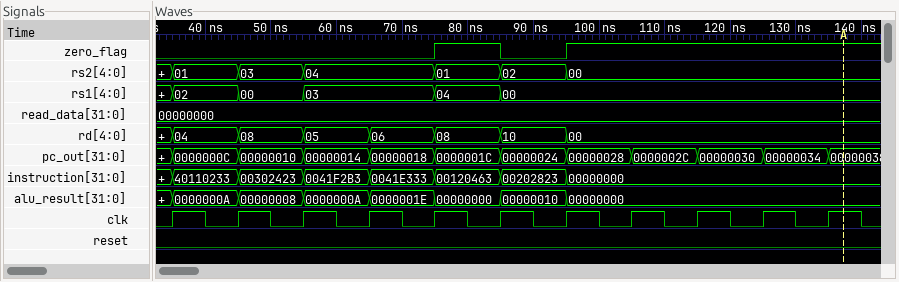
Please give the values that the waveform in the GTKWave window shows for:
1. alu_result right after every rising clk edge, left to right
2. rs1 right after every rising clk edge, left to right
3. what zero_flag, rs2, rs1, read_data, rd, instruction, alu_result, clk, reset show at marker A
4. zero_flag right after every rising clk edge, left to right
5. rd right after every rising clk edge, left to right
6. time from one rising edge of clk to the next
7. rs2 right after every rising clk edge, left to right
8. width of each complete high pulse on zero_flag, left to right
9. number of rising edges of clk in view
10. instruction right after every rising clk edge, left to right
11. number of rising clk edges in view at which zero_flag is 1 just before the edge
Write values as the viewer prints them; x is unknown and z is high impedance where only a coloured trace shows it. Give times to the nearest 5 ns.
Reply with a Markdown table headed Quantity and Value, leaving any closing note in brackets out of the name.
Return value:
| Quantity | Value |
|---|---|
| alu_result right after every rising clk edge, left to right | 0000000A, 00000008, 0000000A, 0000001E, 00000000, 00000010, 00000000, 00000000, 00000000, 00000000, 00000000 |
| rs1 right after every rising clk edge, left to right | 02, 00, 03, 03, 04, 00, 00, 00, 00, 00, 00 |
| what zero_flag, rs2, rs1, read_data, rd, instruction, alu_result, clk, reset show at marker A | zero_flag=1, rs2=00, rs1=00, read_data=00000000, rd=00, instruction=00000000, alu_result=00000000, clk=1, reset=0 |
| zero_flag right after every rising clk edge, left to right | 0 0 0 0 1 0 1 1 1 1 1 |
| rd right after every rising clk edge, left to right | 04, 08, 05, 06, 08, 10, 00, 00, 00, 00, 00 |
| time from one rising edge of clk to the next | 10 ns |
| rs2 right after every rising clk edge, left to right | 01, 03, 04, 04, 01, 02, 00, 00, 00, 00, 00 |
| width of each complete high pulse on zero_flag, left to right | 10 ns |
| number of rising edges of clk in view | 11 |
| instruction right after every rising clk edge, left to right | 40110233, 00302423, 0041F2B3, 0041E333, 00120463, 00202823, 00000000, 00000000, 00000000, 00000000, 00000000 |
| number of rising clk edges in view at which zero_flag is 1 just before the edge | 5 |
